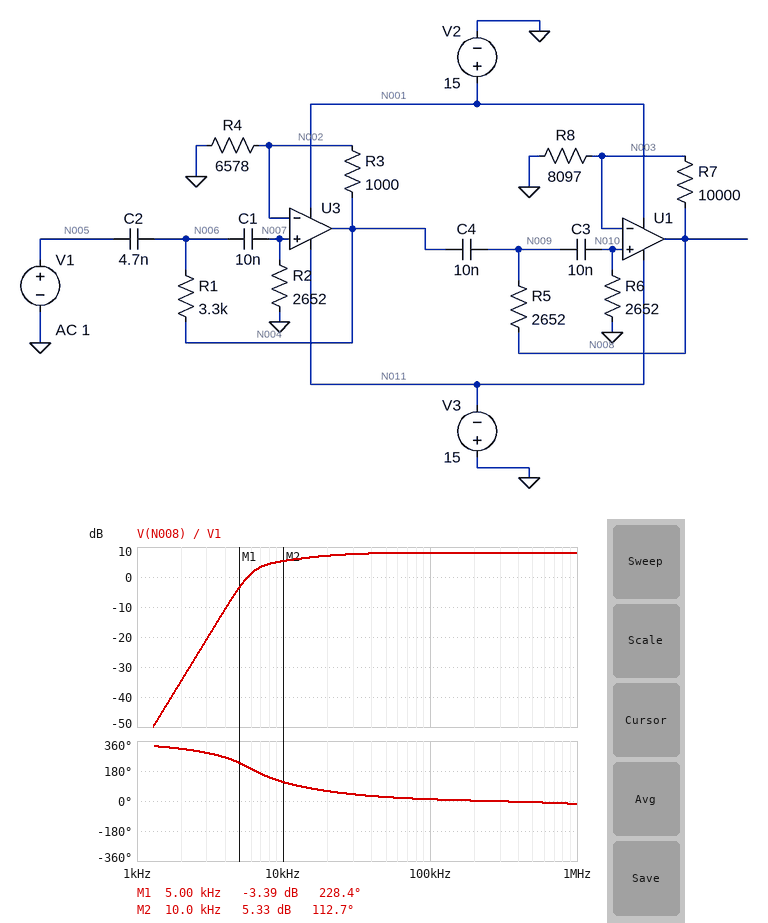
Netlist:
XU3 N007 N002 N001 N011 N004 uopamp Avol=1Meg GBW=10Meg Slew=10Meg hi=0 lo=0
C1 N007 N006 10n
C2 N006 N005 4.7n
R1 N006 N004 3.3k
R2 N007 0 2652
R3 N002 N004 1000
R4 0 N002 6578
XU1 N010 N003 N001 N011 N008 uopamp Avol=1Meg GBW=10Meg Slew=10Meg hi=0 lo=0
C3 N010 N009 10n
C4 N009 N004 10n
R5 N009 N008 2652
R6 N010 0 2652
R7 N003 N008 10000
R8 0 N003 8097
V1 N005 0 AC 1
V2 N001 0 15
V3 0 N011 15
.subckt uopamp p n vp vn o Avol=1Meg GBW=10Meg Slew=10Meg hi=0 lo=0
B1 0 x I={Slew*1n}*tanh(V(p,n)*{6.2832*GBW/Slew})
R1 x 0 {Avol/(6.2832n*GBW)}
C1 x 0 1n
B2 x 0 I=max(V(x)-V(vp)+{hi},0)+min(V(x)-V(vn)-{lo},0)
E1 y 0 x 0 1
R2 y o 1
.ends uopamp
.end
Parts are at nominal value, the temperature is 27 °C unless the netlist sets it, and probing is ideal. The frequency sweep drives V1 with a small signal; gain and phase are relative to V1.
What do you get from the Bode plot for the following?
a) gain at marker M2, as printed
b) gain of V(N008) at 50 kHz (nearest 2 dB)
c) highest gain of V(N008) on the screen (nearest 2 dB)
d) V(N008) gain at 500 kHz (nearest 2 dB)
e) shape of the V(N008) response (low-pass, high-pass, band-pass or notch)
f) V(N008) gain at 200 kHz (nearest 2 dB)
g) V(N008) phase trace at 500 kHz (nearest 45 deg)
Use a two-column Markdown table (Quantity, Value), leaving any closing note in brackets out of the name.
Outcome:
| Quantity | Value |
|---|---|
| gain at marker M2, as printed | 5.33 dB |
| gain of V(N008) at 50 kHz | 8 dB |
| highest gain of V(N008) on the screen | 8 dB |
| V(N008) gain at 500 kHz | 8 dB |
| shape of the V(N008) response | high-pass |
| V(N008) gain at 200 kHz | 8 dB |
| V(N008) phase trace at 500 kHz | 0 deg |
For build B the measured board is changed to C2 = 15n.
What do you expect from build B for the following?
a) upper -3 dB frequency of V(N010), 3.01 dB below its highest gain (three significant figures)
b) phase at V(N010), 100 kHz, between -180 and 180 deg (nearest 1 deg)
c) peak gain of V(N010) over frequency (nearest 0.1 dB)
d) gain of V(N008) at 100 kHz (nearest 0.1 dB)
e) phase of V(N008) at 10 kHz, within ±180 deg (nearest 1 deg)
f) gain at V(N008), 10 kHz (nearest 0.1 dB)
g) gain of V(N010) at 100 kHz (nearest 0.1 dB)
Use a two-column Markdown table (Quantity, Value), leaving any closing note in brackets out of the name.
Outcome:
| Quantity | Value |
|---|---|
| upper -3 dB frequency of V(N010), 3.01 dB below its highest gain | 8.40 MHz |
| phase at V(N010), 100 kHz, between -180 and 180 deg | 7 deg |
| peak gain of V(N010) over frequency | 1.4 dB |
| gain of V(N008) at 100 kHz | 8.2 dB |
| phase of V(N008) at 10 kHz, within ±180 deg | 85 deg |
| gain at V(N008), 10 kHz | 8.3 dB |
| gain of V(N010) at 100 kHz | 1.2 dB |
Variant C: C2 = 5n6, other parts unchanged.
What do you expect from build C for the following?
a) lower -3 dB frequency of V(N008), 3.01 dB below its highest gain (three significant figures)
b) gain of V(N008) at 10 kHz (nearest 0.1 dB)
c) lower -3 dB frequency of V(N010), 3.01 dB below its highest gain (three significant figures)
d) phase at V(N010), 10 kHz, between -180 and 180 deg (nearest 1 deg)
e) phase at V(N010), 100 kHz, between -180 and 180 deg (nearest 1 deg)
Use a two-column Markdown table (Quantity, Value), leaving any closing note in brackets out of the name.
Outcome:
| Quantity | Value |
|---|---|
| lower -3 dB frequency of V(N008), 3.01 dB below its highest gain | 7.79 kHz |
| gain of V(N008) at 10 kHz | 6.1 dB |
| lower -3 dB frequency of V(N010), 3.01 dB below its highest gain | 7.81 kHz |
| phase at V(N010), 10 kHz, between -180 and 180 deg | 108 deg |
| phase at V(N010), 100 kHz, between -180 and 180 deg | 11 deg |
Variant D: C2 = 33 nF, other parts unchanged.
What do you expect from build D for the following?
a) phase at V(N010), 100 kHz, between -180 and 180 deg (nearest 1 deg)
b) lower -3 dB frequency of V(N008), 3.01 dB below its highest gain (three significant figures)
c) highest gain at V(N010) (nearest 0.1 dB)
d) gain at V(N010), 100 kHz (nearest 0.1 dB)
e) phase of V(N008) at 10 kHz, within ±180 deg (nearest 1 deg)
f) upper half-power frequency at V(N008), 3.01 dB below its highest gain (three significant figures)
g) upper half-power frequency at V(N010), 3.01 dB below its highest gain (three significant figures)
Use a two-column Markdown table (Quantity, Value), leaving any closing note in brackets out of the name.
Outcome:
| Quantity | Value |
|---|---|
| phase at V(N010), 100 kHz, between -180 and 180 deg | 6 deg |
| lower -3 dB frequency of V(N008), 3.01 dB below its highest gain | 5.54 kHz |
| highest gain at V(N010) | 1.9 dB |
| gain at V(N010), 100 kHz | 1.2 dB |
| phase of V(N008) at 10 kHz, within ±180 deg | 75 deg |
| upper half-power frequency at V(N008), 3.01 dB below its highest gain | 3.18 MHz |
| upper half-power frequency at V(N010), 3.01 dB below its highest gain | 7.33 MHz |
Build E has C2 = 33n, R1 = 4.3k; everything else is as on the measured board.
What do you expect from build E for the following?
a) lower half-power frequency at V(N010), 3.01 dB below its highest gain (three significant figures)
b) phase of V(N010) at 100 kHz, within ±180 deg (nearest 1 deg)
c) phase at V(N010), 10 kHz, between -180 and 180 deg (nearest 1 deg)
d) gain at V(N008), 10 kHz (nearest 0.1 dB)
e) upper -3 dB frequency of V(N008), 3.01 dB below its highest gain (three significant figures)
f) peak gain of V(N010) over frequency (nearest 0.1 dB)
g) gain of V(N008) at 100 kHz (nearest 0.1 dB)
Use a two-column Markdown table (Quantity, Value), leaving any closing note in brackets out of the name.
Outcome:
| Quantity | Value |
|---|---|
| lower half-power frequency at V(N010), 3.01 dB below its highest gain | 5.55 kHz |
| phase of V(N010) at 100 kHz, within ±180 deg | 6 deg |
| phase at V(N010), 10 kHz, between -180 and 180 deg | 75 deg |
| gain at V(N008), 10 kHz | 8.6 dB |
| upper -3 dB frequency of V(N008), 3.01 dB below its highest gain | 3.32 MHz |
| peak gain of V(N010) over frequency | 1.7 dB |
| gain of V(N008) at 100 kHz | 8.2 dB |
